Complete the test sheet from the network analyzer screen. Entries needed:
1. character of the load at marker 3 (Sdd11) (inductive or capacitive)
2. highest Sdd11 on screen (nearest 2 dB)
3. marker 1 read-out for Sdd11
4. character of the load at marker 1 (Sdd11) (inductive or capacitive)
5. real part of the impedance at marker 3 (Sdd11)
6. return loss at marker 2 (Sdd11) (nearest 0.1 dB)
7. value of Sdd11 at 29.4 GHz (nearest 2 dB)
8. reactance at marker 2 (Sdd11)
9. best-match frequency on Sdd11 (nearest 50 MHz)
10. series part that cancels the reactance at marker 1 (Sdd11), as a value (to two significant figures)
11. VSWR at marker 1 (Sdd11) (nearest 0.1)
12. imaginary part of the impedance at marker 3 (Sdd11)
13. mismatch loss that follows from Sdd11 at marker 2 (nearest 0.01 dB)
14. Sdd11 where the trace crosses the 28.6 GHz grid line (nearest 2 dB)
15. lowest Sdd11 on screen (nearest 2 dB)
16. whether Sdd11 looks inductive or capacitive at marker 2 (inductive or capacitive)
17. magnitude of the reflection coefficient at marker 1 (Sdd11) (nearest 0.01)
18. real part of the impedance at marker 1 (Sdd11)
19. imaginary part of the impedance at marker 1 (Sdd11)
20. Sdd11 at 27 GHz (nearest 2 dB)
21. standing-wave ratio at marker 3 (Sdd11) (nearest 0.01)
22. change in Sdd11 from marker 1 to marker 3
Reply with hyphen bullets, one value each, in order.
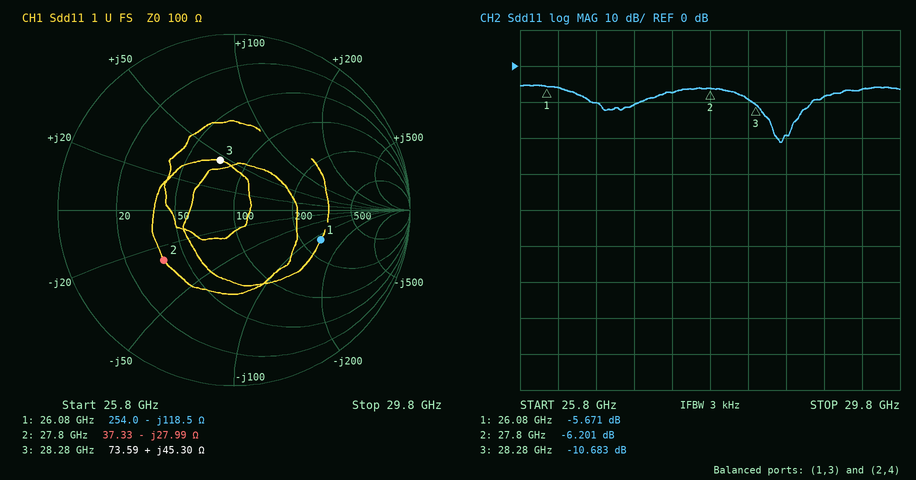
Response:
- inductive
- -6 dB
- -5.671 dB
- capacitive
- 73.59 Ω
- 6.2 dB
- -6 dB
- -27.99 Ω
- 28.55 GHz
- 720 pH
- 3.2
- +45.30 Ω
- 1.19 dB
- -20 dB
- -22 dB
- capacitive
- 0.52
- 254.0 Ω
- -118.5 Ω
- -10 dB
- 1.83
- -5.012 dB
